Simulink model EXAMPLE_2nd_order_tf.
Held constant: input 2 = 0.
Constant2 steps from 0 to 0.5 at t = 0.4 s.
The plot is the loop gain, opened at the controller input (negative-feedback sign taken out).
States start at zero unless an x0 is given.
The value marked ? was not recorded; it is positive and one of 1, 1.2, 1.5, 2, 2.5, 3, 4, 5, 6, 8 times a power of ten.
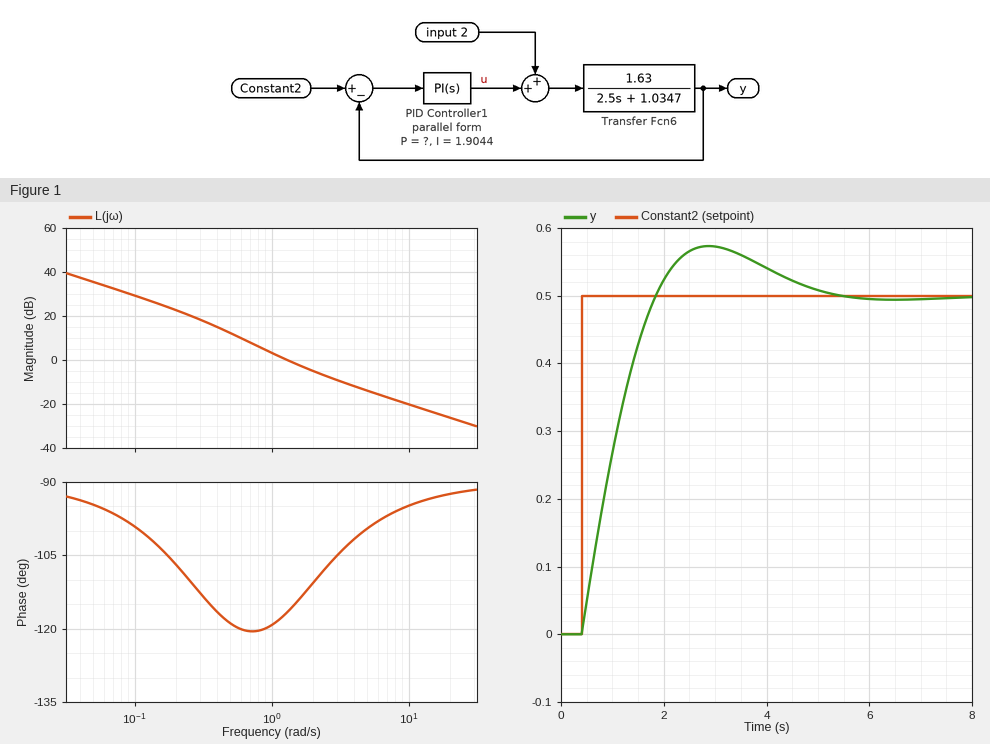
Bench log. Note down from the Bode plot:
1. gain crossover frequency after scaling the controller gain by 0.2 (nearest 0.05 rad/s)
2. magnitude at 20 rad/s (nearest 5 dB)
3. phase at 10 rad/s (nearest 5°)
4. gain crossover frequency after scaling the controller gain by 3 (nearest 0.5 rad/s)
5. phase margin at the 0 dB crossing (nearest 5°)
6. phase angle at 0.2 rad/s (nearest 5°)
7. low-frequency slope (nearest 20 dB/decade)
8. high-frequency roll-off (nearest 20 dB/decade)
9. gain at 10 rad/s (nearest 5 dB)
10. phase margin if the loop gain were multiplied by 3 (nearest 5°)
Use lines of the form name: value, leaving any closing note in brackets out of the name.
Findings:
gain crossover frequency after scaling the controller gain by 0.2: 0.45 rad/s
magnitude at 20 rad/s: -25 dB
phase at 10 rad/s: -95°
gain crossover frequency after scaling the controller gain by 3: 3.0 rad/s
phase margin at the 0 dB crossing: 65°
phase angle at 0.2 rad/s: -105°
low-frequency slope: -20 dB/decade
high-frequency roll-off: -20 dB/decade
gain at 10 rad/s: -20 dB
phase margin if the loop gain were multiplied by 3: 75°
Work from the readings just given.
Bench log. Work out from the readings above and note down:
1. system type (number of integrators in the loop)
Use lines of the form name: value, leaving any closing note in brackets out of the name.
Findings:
system type: 1
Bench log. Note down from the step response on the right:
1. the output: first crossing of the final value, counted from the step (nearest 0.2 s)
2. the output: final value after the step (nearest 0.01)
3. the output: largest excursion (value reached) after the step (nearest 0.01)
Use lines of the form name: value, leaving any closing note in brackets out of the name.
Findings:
the output: first crossing of the final value, counted from the step: 1.4 s
the output: final value after the step: 0.50
the output: largest excursion (value reached) after the step: 0.57
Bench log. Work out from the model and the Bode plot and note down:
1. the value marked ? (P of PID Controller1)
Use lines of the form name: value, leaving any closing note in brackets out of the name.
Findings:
the value marked ?: 1.5
